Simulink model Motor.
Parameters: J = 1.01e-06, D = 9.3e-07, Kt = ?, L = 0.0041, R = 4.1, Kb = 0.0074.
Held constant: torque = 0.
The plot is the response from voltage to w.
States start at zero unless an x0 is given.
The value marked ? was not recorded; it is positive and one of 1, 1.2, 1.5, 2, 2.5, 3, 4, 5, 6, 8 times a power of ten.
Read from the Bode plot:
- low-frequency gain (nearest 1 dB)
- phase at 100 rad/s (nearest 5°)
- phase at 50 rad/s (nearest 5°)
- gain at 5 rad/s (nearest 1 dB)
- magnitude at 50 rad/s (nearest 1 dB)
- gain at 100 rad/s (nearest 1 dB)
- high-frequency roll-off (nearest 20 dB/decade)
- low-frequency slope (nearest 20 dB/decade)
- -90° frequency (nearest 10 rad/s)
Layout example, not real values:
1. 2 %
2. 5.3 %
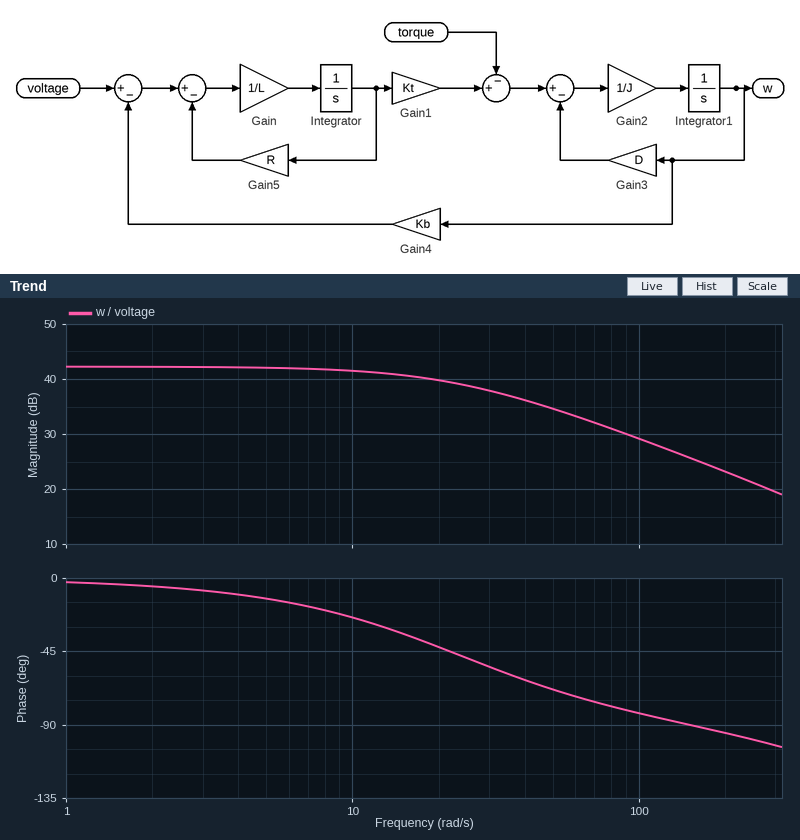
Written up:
1. 42 dB
2. -85°
3. -70°
4. 42 dB
5. 35 dB
6. 29 dB
7. -20 dB/decade
8. 0 dB/decade
9. 150 rad/s
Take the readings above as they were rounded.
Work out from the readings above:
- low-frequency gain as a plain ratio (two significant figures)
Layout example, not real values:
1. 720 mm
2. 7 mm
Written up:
1. 130
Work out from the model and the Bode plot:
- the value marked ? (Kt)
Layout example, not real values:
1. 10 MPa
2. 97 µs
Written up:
1. 0.012
